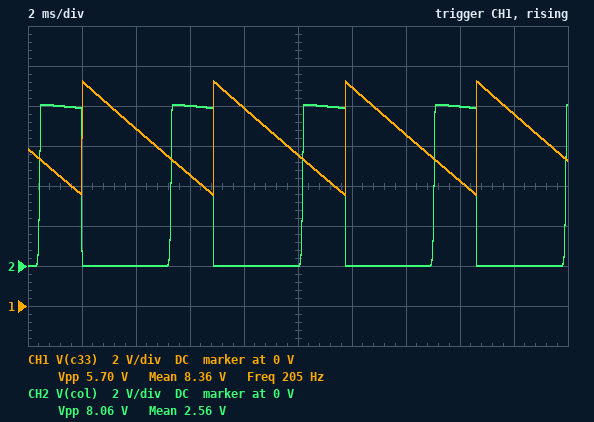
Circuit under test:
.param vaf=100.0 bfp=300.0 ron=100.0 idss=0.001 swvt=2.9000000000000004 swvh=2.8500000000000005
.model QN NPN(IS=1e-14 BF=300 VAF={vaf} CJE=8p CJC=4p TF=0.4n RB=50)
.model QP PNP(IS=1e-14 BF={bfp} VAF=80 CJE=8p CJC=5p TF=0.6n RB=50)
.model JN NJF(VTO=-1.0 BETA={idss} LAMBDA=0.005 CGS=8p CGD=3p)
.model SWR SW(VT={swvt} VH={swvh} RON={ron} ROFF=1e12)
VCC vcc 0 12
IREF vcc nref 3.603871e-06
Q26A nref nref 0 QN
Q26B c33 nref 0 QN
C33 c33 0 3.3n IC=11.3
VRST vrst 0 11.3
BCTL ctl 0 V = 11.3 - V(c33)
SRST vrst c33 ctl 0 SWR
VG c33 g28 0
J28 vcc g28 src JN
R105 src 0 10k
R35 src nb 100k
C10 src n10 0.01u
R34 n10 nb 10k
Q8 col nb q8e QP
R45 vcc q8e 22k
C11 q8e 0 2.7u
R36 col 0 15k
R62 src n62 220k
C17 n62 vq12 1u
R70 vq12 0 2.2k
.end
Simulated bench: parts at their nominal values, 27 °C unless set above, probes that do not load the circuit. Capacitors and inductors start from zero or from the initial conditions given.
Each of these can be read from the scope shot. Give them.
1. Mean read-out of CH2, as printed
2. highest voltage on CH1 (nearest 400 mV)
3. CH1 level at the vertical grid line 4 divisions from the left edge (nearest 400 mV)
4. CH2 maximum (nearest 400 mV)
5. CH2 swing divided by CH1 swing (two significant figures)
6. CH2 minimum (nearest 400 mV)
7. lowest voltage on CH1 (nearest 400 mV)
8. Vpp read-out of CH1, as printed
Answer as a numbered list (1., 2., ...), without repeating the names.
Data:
1. 2.56 V
2. 11.2 V
3. 10.0 V
4. 8.0 V
5. 1.4
6. 0 V
7. 5.6 V
8. 5.70 V
